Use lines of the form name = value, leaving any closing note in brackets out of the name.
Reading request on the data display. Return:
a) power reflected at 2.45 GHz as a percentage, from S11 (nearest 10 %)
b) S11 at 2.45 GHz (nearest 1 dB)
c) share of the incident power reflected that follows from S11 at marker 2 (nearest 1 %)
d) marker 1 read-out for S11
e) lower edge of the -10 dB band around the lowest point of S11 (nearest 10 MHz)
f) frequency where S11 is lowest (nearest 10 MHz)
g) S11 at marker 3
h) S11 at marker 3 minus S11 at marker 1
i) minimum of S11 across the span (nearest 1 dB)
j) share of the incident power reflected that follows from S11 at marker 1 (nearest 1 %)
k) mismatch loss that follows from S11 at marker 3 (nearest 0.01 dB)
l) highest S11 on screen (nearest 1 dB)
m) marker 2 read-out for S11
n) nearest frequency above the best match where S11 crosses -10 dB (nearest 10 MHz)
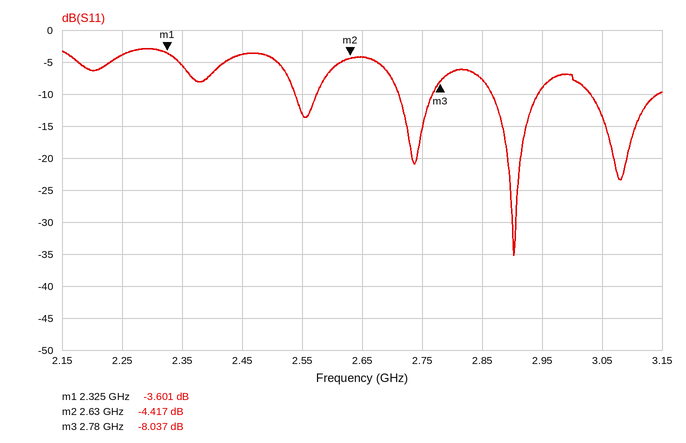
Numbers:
power reflected at 2.45 GHz as a percentage, from S11 = 40 %
S11 at 2.45 GHz = -4 dB
share of the incident power reflected that follows from S11 at marker 2 = 36 %
marker 1 read-out for S11 = -3.601 dB
lower edge of the -10 dB band around the lowest point of S11 = 2.87 GHz
frequency where S11 is lowest = 2.90 GHz
S11 at marker 3 = -8.037 dB
S11 at marker 3 minus S11 at marker 1 = -4.436 dB
minimum of S11 across the span = -35 dB
share of the incident power reflected that follows from S11 at marker 1 = 44 %
mismatch loss that follows from S11 at marker 3 = 0.74 dB
highest S11 on screen = -3 dB
marker 2 read-out for S11 = -4.417 dB
nearest frequency above the best match where S11 crosses -10 dB = 2.94 GHz
